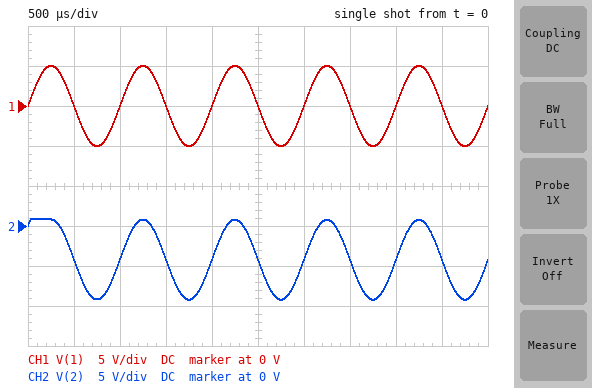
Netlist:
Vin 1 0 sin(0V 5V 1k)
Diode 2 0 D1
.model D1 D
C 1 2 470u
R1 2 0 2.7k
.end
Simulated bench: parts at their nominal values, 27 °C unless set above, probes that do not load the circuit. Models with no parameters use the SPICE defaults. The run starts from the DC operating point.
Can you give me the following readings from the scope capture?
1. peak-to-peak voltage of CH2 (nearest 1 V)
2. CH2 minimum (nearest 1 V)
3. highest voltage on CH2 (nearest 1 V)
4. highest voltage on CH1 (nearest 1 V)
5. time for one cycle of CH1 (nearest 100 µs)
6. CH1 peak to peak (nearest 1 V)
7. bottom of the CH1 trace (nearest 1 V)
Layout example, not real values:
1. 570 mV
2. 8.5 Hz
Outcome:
1. 10 V
2. -9 V
3. 1 V
4. 5 V
5. 1.0 ms
6. 10 V
7. -5 V
